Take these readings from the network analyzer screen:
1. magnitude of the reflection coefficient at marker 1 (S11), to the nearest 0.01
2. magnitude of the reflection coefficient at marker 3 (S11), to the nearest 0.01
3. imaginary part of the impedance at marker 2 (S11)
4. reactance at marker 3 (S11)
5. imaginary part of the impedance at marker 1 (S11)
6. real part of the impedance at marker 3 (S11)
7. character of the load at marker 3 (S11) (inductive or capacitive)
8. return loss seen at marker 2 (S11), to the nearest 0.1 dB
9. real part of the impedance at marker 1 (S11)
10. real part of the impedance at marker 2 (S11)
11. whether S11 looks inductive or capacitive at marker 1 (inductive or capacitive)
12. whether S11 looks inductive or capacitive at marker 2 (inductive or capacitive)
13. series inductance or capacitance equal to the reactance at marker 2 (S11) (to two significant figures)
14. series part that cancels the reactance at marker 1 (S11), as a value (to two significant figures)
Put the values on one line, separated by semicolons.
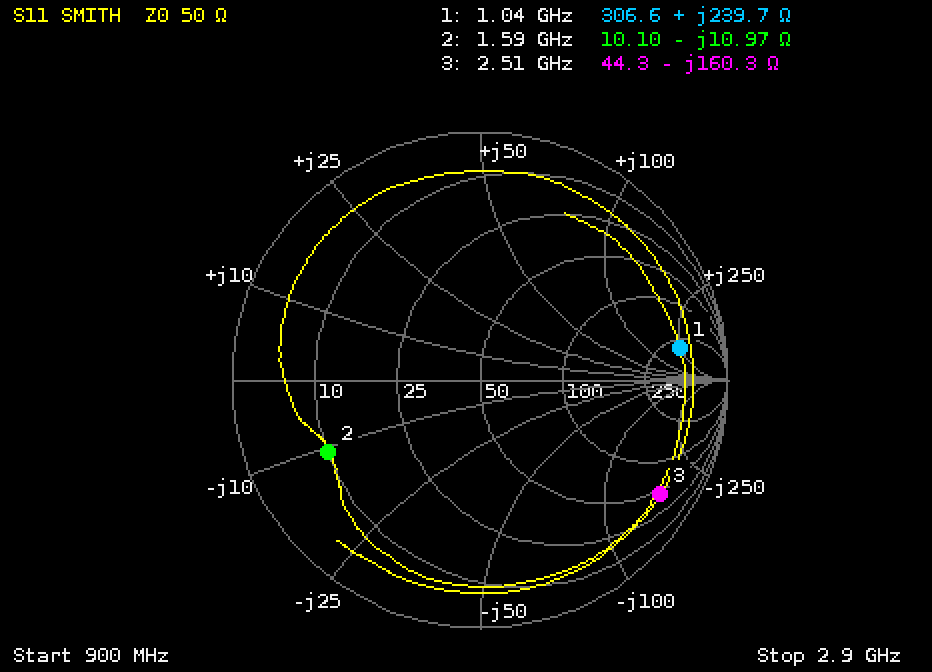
0.82; 0.86; -10.97 Ω; -160.3 Ω; +239.7 Ω; 44.3 Ω; capacitive; 3.4 dB; 306.6 Ω; 10.10 Ω; inductive; capacitive; 9.1 pF; 640 fF
